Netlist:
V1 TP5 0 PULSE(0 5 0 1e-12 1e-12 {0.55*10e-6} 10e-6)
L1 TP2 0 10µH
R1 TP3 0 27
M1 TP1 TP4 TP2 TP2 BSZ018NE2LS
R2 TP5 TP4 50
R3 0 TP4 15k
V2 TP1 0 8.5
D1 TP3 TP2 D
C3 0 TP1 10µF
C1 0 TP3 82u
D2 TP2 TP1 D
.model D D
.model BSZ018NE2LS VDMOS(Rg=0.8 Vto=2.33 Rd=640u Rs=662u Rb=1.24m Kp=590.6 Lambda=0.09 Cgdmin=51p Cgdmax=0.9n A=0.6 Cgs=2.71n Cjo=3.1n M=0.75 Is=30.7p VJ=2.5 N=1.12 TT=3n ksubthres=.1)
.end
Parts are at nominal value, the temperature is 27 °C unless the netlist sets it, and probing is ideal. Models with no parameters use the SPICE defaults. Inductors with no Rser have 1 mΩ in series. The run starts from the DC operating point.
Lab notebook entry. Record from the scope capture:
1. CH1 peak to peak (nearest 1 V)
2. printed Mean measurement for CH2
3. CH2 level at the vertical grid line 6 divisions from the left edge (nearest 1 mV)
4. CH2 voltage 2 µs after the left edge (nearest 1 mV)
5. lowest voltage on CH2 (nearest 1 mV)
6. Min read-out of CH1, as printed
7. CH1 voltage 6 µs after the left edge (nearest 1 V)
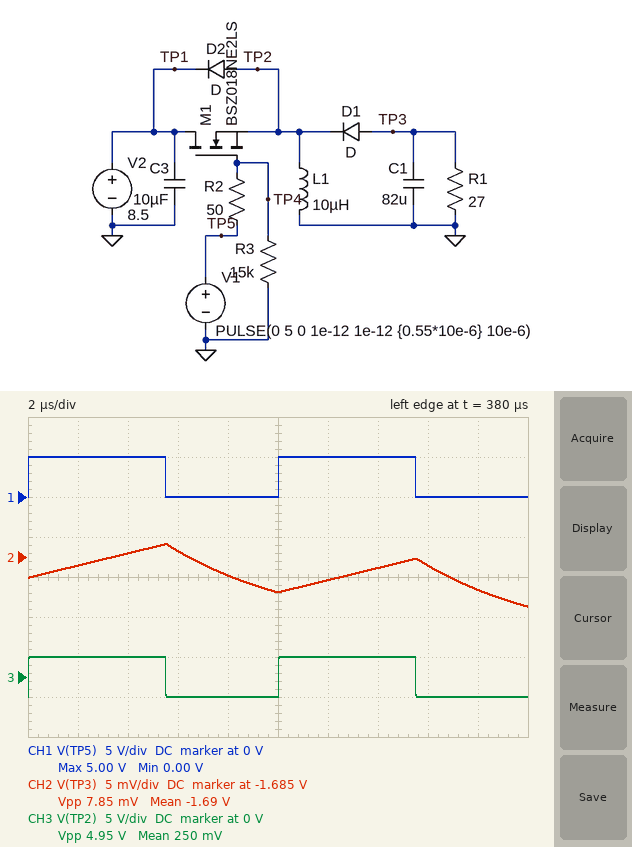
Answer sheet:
5 V
-1.69 V
-1.688 V
-1.686 V
-1.691 V
0.00 V
0 V
